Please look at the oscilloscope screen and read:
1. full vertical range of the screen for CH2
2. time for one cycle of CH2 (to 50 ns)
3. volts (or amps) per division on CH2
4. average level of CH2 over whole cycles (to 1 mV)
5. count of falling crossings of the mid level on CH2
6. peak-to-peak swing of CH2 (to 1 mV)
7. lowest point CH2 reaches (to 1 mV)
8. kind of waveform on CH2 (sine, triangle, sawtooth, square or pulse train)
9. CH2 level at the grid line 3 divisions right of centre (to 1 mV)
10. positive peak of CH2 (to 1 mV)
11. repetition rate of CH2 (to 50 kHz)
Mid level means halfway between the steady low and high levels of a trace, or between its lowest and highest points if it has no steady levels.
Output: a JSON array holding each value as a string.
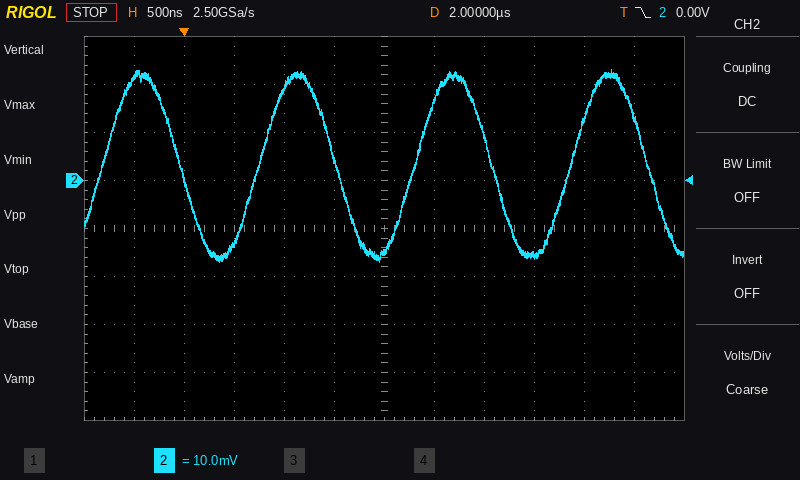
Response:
["80 mV", "1.55 µs", "10 mV", "3 mV", "4", "40 mV", "-17 mV", "sine", "-16 mV", "23 mV", "650 kHz"]
